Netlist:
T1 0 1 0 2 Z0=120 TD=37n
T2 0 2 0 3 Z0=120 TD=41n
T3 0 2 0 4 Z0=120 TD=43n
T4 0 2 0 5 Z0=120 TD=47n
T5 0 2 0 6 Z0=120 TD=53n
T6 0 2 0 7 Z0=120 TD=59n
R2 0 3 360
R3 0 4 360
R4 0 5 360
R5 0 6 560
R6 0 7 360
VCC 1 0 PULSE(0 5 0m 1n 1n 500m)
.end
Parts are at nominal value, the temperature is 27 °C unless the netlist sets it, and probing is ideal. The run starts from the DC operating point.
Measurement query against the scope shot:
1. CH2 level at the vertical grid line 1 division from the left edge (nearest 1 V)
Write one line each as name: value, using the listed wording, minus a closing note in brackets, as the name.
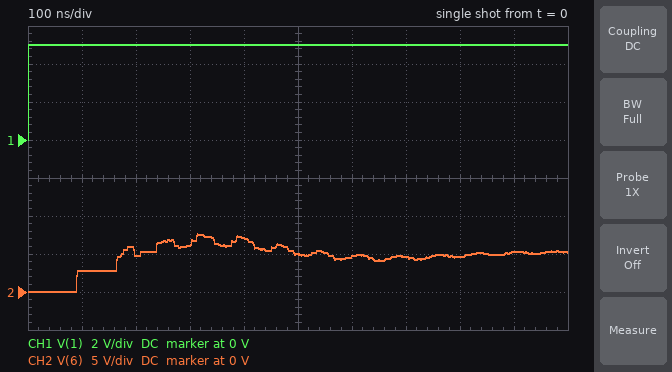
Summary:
CH2 level at the vertical grid line 1 division from the left edge: 3 V
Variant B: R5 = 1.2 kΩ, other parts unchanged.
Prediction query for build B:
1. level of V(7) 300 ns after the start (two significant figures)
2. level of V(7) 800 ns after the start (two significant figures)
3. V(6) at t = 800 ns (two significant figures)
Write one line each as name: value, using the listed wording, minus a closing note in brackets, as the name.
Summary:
level of V(7) 300 ns after the start: 6.9 V
level of V(7) 800 ns after the start: 4.8 V
V(6) at t = 800 ns: 4.4 V
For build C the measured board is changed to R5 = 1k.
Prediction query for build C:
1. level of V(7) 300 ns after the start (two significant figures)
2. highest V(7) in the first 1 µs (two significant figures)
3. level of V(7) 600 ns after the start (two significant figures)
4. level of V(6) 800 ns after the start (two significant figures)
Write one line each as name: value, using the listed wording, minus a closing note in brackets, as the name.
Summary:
level of V(7) 300 ns after the start: 6.9 V
highest V(7) in the first 1 µs: 7.3 V
level of V(7) 600 ns after the start: 4.3 V
level of V(6) 800 ns after the start: 4.4 V
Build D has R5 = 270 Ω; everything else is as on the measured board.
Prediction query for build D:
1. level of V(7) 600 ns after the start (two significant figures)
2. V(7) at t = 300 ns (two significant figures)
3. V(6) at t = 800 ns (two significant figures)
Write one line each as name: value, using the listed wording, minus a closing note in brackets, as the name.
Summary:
level of V(7) 600 ns after the start: 4.6 V
V(7) at t = 300 ns: 6.1 V
V(6) at t = 800 ns: 4.8 V
